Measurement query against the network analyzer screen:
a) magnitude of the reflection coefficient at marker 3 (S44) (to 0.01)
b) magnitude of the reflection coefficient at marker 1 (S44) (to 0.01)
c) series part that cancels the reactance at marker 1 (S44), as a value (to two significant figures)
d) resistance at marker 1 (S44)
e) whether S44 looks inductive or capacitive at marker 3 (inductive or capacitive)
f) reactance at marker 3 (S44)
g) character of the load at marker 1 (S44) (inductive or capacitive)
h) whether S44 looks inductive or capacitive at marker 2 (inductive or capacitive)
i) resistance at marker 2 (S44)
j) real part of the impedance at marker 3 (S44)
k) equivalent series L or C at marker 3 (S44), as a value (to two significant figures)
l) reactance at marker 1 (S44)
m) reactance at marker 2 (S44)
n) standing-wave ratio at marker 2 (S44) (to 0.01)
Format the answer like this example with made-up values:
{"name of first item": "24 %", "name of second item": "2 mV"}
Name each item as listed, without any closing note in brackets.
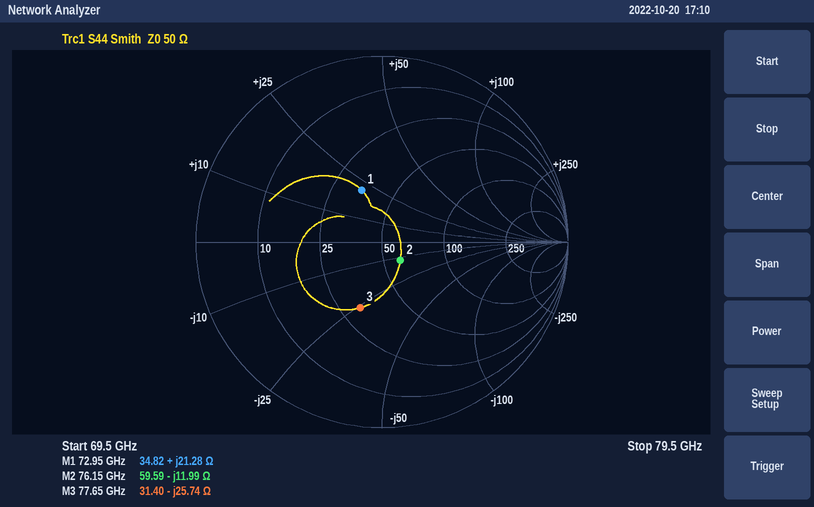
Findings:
{"magnitude of the reflection coefficient at marker 3 (S44)": "0.37", "magnitude of the reflection coefficient at marker 1 (S44)": "0.30", "series part that cancels the reactance at marker 1 (S44), as a value": "100 fF", "resistance at marker 1": "34.82 Ω", "whether S44 looks inductive or capacitive at marker 3": "capacitive", "reactance at marker 3": "-25.74 Ω", "character of the load at marker 1 (S44)": "inductive", "whether S44 looks inductive or capacitive at marker 2": "capacitive", "resistance at marker 2": "59.59 Ω", "real part of the impedance at marker 3": "31.40 Ω", "equivalent series L or C at marker 3 (S44), as a value": "80 fF", "reactance at marker 1": "+21.28 Ω", "reactance at marker 2": "-11.99 Ω", "standing-wave ratio at marker 2 (S44)": "1.32"}
